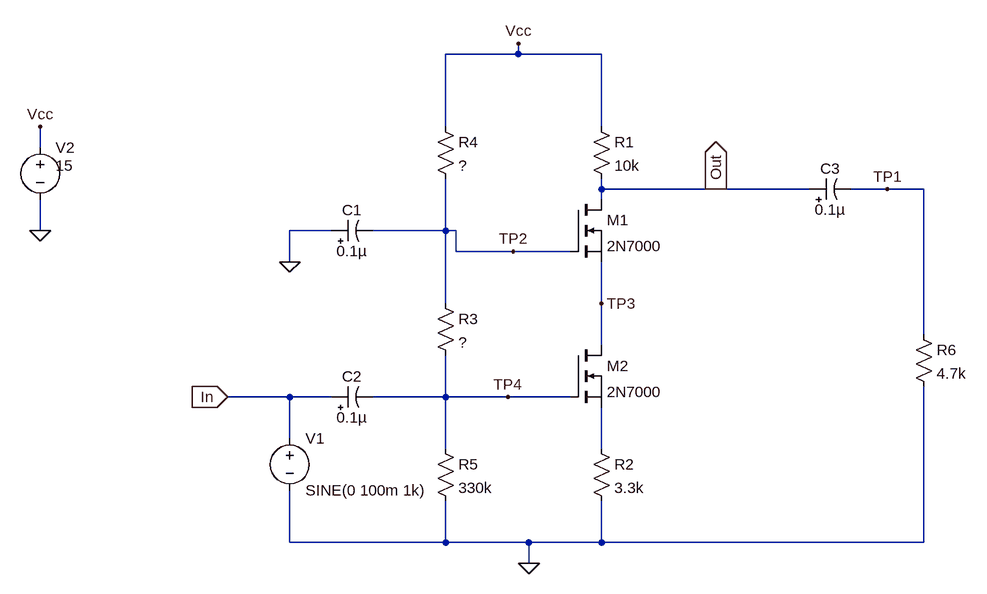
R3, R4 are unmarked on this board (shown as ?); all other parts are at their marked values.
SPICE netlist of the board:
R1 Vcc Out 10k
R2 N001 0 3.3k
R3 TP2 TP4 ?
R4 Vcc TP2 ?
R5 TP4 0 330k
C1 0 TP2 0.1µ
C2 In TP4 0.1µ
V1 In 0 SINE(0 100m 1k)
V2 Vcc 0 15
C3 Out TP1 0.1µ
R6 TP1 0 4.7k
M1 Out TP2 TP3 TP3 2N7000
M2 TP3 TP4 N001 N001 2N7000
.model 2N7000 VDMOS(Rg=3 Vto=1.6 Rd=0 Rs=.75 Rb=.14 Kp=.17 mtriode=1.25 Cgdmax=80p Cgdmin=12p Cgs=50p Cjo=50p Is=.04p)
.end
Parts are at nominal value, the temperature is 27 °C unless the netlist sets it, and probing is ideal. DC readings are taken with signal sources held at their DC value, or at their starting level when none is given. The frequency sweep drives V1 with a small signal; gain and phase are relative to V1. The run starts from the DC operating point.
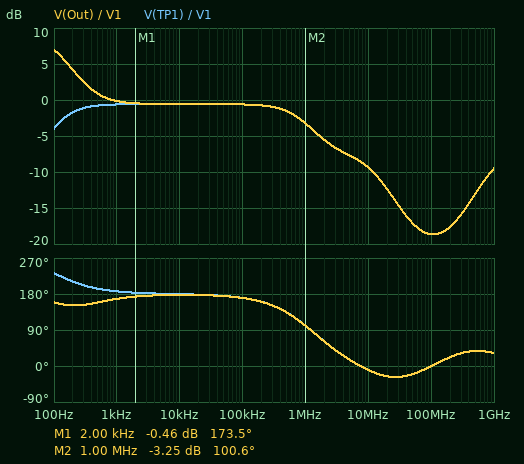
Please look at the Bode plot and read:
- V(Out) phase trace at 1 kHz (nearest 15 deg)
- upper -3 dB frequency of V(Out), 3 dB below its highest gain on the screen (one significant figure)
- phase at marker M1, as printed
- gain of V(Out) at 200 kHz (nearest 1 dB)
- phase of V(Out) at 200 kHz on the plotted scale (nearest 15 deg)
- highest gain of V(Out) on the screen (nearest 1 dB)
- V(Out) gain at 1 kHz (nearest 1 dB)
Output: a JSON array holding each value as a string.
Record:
["165 deg", "200 Hz", "173.5 deg", "-1 dB", "165 deg", "7 dB", "0 dB"]
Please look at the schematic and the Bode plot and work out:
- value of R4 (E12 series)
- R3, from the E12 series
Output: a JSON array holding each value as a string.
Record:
["560 kΩ", "390 kΩ"]
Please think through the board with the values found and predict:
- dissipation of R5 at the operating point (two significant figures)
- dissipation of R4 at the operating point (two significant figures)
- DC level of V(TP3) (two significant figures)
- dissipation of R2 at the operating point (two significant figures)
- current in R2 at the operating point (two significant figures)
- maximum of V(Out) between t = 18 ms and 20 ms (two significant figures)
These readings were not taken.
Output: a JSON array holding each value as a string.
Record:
["45 µW", "77 µW", "6.8 V", "1.5 mW", "680 µA", "8.3 V"]
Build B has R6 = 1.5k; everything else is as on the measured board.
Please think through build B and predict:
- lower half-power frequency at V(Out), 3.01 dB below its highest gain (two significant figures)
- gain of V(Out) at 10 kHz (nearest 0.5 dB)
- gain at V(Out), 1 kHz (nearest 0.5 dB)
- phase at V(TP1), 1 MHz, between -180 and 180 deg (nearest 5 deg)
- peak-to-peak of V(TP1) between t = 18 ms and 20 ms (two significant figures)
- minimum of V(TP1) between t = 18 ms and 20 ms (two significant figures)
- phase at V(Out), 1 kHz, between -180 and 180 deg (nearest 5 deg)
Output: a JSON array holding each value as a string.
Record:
["7.9 Hz", "-8.5 dB", "-5.0 dB", "125 deg", "76 mV", "-38 mV", "140 deg"]
